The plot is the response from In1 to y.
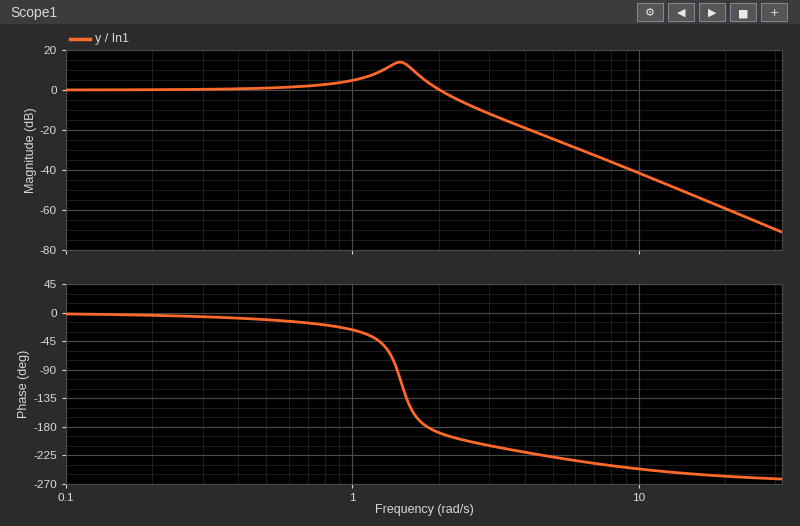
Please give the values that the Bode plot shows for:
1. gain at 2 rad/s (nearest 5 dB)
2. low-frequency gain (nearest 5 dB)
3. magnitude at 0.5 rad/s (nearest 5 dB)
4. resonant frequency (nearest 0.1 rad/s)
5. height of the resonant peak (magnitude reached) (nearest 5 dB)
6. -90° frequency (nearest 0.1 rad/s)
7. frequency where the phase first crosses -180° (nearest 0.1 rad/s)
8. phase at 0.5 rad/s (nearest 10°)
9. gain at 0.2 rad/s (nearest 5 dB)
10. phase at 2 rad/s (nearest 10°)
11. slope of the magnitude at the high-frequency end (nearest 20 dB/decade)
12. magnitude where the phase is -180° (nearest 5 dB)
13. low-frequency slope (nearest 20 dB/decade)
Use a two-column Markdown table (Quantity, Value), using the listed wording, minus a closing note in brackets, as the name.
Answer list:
| Quantity | Value |
|---|---|
| gain at 2 rad/s | 0 dB |
| low-frequency gain | 0 dB |
| magnitude at 0.5 rad/s | 0 dB |
| resonant frequency | 1.5 rad/s |
| height of the resonant peak (magnitude reached) | 15 dB |
| -90° frequency | 1.4 rad/s |
| frequency where the phase first crosses -180° | 1.8 rad/s |
| phase at 0.5 rad/s | -10° |
| gain at 0.2 rad/s | 0 dB |
| phase at 2 rad/s | -190° |
| slope of the magnitude at the high-frequency end | -60 dB/decade |
| magnitude where the phase is -180° | 5 dB |
| low-frequency slope | 0 dB/decade |
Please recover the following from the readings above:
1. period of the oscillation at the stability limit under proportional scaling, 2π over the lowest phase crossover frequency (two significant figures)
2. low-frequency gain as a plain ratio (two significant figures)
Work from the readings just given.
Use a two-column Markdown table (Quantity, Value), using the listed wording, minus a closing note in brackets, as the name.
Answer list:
| Quantity | Value |
|---|---|
| period of the oscillation at the stability limit under proportional scaling, 2π over the lowest phase crossover frequency | 3.5 s |
| low-frequency gain as a plain ratio | 1.0 |
